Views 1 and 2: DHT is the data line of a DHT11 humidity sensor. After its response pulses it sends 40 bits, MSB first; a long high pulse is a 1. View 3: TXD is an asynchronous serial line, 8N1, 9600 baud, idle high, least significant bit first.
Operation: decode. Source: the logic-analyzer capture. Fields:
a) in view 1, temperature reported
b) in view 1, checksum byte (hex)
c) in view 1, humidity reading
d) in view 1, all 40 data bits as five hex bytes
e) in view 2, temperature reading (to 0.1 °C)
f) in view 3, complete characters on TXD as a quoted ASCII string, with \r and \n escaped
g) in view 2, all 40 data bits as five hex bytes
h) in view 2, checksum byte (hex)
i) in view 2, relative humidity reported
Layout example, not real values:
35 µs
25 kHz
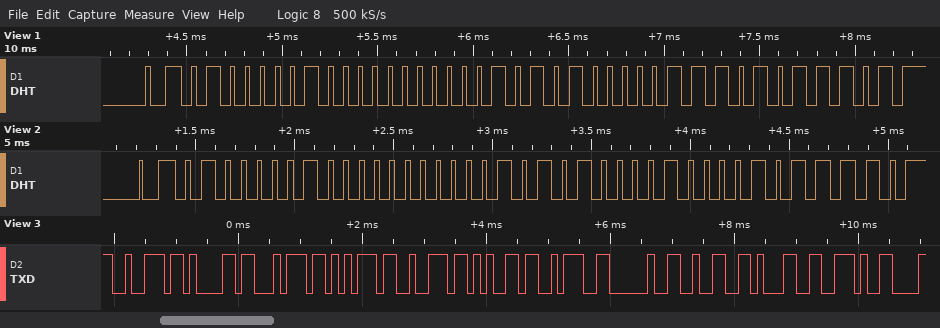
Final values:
21.7 °C
0x5D
65 %
41 00 15 07 5D
21.8 °C
"rature: 21."
41 00 15 08 5E
0x5E
65 %
